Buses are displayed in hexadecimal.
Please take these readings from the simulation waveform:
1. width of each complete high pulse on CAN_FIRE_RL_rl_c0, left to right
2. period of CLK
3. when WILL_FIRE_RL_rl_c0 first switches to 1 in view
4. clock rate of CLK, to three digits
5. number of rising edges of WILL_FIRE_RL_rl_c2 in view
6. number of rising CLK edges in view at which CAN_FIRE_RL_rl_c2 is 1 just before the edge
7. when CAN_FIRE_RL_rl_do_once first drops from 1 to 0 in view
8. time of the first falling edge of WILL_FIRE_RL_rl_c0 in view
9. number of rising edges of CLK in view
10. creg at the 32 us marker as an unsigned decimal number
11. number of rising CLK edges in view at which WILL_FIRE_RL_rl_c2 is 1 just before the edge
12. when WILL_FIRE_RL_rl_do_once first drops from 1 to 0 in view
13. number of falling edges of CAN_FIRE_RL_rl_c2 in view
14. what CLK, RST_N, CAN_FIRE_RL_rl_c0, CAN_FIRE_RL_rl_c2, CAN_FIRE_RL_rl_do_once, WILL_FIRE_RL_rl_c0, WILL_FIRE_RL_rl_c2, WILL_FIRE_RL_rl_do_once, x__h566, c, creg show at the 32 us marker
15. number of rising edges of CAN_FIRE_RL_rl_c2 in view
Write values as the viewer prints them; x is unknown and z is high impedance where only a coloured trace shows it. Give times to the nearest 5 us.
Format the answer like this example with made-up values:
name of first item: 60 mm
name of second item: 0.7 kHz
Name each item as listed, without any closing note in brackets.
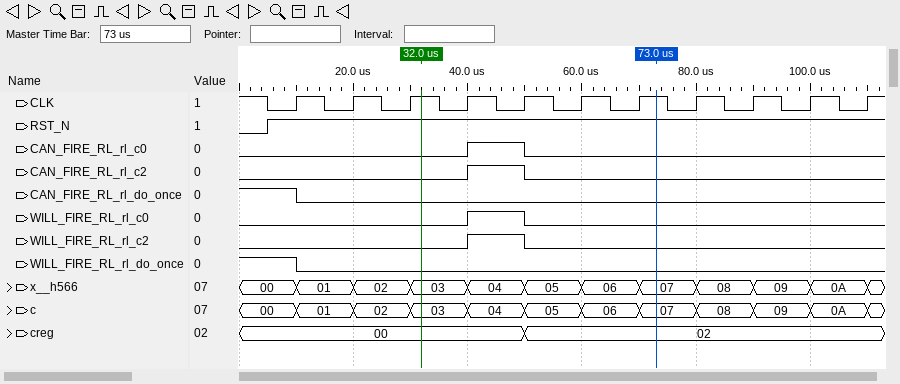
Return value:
width of each complete high pulse on CAN_FIRE_RL_rl_c0, left to right: 10 us
period of CLK: 10 us
when WILL_FIRE_RL_rl_c0 first switches to 1 in view: 40 us
clock rate of CLK, to three digits: 100 kHz
number of rising edges of WILL_FIRE_RL_rl_c2 in view: 1
number of rising CLK edges in view at which CAN_FIRE_RL_rl_c2 is 1 just before the edge: 1
when CAN_FIRE_RL_rl_do_once first drops from 1 to 0 in view: 10 us
time of the first falling edge of WILL_FIRE_RL_rl_c0 in view: 50 us
number of rising edges of CLK in view: 11
creg at the 32 us marker as an unsigned decimal number: 0
number of rising CLK edges in view at which WILL_FIRE_RL_rl_c2 is 1 just before the edge: 1
when WILL_FIRE_RL_rl_do_once first drops from 1 to 0 in view: 10 us
number of falling edges of CAN_FIRE_RL_rl_c2 in view: 1
what CLK, RST_N, CAN_FIRE_RL_rl_c0, CAN_FIRE_RL_rl_c2, CAN_FIRE_RL_rl_do_once, WILL_FIRE_RL_rl_c0, WILL_FIRE_RL_rl_c2, WILL_FIRE_RL_rl_do_once, x__h566, c, creg show at the 32 us marker: CLK=1, RST_N=1, CAN_FIRE_RL_rl_c0=0, CAN_FIRE_RL_rl_c2=0, CAN_FIRE_RL_rl_do_once=0, WILL_FIRE_RL_rl_c0=0, WILL_FIRE_RL_rl_c2=0, WILL_FIRE_RL_rl_do_once=0, x__h566=03, c=03, creg=00
number of rising edges of CAN_FIRE_RL_rl_c2 in view: 1
